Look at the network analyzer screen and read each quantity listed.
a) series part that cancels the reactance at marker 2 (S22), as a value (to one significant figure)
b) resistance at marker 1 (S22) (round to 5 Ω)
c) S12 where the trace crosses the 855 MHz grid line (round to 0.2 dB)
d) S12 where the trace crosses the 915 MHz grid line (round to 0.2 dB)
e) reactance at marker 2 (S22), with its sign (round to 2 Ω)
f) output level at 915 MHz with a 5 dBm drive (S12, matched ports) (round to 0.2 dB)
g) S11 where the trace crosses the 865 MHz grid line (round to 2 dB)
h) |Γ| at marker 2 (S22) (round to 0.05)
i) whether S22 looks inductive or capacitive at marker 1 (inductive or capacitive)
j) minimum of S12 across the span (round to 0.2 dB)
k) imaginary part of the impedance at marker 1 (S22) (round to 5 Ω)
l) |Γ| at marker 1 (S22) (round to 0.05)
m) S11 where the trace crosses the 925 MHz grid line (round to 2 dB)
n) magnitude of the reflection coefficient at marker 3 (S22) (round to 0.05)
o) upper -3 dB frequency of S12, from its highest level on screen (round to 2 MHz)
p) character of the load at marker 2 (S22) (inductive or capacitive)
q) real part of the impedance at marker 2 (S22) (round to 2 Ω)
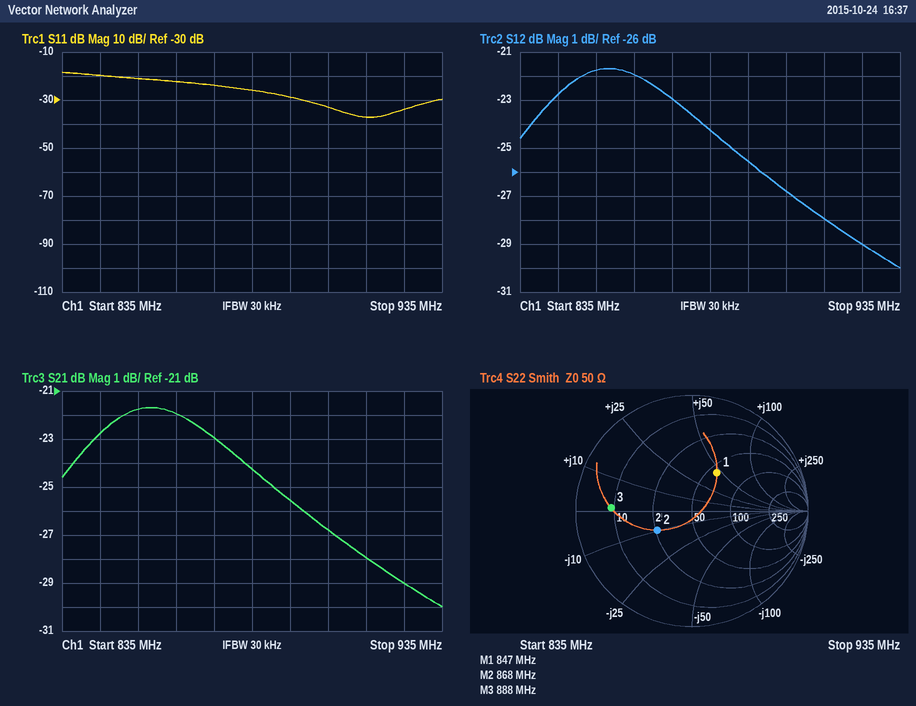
2 nH
60 Ω
-21.8 dB
-28.0 dB
-10 Ω
-23.0 dBm
-22 dB
0.35
inductive
-30.0 dB
+45 Ω
0.40
-34 dB
0.70
888 MHz
capacitive
26 Ω
